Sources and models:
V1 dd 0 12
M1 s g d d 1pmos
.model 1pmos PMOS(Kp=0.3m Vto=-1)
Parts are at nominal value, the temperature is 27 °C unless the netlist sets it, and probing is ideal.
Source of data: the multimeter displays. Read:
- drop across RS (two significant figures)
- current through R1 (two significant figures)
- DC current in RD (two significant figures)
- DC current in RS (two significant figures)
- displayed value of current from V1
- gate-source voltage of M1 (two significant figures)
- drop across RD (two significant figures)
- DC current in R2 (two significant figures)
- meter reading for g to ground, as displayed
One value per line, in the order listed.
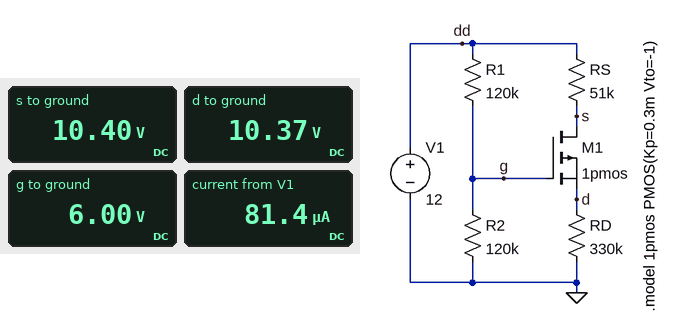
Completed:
1.6 V
50 µA
31 µA
31 µA
81.4 µA
-4.4 V
10 V
50 µA
6.00 V
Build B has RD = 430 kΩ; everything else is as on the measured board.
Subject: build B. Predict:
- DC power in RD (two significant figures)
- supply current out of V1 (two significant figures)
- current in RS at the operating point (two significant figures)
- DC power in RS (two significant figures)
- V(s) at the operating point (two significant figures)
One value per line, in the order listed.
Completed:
270 µW
75 µA
25 µA
32 µW
11 V
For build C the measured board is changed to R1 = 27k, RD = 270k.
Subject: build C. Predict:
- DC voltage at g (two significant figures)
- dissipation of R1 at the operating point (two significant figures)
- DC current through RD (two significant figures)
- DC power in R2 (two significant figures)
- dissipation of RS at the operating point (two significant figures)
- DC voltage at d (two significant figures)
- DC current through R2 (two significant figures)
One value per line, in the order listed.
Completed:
9.8 V
180 µW
36 µA
800 µW
65 µW
9.6 V
82 µA
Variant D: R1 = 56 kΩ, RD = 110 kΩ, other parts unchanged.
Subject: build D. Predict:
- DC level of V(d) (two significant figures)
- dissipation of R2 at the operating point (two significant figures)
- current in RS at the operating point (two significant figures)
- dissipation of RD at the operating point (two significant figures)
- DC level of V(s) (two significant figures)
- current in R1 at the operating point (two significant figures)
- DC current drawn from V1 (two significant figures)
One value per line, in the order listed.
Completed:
7.8 V
560 µW
71 µA
550 µW
8.4 V
68 µA
140 µA
